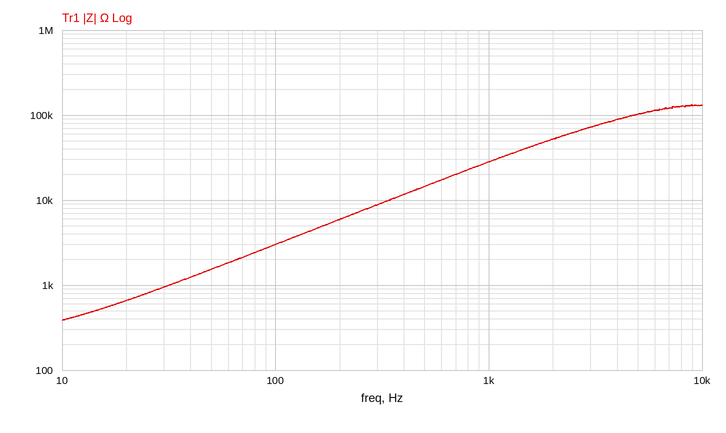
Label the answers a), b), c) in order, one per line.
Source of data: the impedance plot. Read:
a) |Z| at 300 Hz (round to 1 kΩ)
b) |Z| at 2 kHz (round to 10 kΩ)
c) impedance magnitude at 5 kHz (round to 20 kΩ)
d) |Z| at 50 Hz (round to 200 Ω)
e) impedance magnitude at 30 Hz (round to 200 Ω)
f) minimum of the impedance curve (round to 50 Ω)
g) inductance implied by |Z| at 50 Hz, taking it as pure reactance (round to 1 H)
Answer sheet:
a) 9 kΩ
b) 50 kΩ
c) 100 kΩ
d) 1.6 kΩ
e) 1.0 kΩ
f) 400 Ω
g) 5 H
